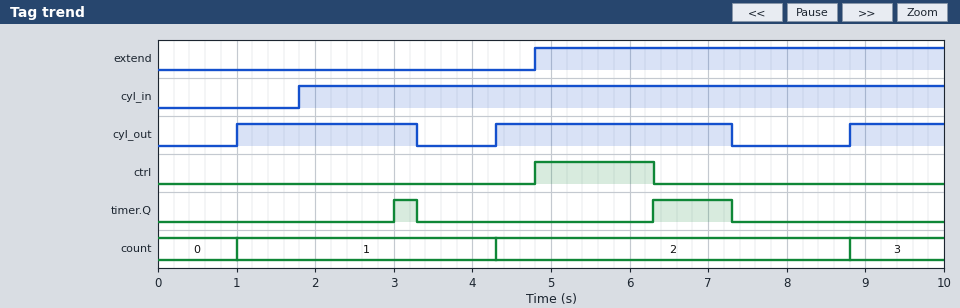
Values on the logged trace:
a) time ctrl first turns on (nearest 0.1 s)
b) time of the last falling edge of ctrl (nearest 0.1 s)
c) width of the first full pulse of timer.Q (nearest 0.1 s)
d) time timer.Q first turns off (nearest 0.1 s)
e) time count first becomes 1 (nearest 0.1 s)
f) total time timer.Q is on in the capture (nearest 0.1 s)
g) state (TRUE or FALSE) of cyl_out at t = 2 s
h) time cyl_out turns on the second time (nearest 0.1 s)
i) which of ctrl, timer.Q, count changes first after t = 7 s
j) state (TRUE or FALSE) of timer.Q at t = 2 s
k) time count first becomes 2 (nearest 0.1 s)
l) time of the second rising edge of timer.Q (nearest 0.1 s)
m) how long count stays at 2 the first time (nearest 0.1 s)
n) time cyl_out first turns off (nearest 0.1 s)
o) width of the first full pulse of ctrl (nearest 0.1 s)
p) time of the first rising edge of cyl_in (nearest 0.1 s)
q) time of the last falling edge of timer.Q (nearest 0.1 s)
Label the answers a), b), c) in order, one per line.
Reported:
a) 4.8 s
b) 6.3 s
c) 0.3 s
d) 3.3 s
e) 1.0 s
f) 1.3 s
g) TRUE
h) 4.3 s
i) timer.Q
j) FALSE
k) 4.3 s
l) 6.3 s
m) 4.5 s
n) 3.3 s
o) 1.5 s
p) 1.8 s
q) 7.3 s
